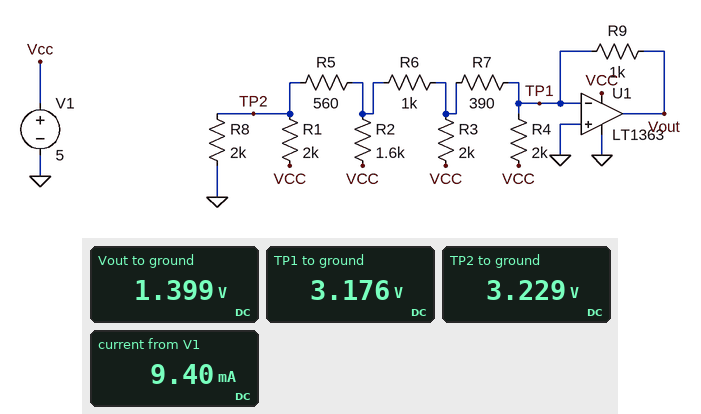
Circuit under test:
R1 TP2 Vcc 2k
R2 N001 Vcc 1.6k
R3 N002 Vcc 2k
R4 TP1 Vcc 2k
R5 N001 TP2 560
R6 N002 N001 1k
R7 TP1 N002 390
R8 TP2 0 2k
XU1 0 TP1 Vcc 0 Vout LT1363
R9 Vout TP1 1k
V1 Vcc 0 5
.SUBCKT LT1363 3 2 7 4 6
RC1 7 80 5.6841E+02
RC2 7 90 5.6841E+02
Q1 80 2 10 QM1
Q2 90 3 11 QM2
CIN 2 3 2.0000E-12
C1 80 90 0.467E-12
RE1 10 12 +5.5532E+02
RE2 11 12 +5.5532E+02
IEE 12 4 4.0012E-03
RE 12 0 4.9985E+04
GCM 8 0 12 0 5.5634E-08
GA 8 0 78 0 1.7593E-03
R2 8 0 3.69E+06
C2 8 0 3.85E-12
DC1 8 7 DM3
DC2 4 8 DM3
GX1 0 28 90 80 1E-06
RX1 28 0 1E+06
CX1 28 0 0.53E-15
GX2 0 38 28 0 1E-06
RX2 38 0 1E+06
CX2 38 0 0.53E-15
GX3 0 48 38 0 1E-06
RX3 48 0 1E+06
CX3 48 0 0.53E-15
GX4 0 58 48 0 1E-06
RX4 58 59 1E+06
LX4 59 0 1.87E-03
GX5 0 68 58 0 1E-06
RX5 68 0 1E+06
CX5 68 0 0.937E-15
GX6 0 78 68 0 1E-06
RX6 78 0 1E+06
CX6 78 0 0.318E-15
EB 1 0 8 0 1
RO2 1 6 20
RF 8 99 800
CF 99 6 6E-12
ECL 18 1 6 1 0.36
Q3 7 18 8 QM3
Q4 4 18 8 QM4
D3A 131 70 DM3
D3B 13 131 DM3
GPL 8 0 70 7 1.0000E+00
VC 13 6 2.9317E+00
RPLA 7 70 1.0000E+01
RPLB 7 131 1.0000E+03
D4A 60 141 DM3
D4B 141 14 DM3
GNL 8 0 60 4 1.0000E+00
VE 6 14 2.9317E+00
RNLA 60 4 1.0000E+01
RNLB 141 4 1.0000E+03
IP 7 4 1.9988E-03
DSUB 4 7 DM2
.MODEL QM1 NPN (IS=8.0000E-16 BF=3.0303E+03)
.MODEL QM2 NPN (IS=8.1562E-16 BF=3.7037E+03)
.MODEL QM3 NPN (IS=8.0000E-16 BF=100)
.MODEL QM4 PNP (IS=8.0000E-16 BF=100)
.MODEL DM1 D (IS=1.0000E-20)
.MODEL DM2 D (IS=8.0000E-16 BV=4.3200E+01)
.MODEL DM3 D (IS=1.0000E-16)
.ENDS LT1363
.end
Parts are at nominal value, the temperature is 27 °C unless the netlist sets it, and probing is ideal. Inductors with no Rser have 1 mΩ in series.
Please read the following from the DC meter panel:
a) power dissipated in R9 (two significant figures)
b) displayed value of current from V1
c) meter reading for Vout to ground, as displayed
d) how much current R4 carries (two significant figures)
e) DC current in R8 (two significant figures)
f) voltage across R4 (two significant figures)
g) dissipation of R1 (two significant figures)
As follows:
3.2 mW
9.40 mA
1.399 V
910 µA
1.6 mA
1.8 V
1.6 mW
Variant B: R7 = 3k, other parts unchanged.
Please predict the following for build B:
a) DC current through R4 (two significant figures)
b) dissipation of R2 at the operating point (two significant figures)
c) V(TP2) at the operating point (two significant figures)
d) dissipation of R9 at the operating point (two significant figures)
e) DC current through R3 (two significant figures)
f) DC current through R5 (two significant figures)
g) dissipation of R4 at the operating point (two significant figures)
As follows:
1.1 mA
840 µW
3.4 V
2.1 mW
510 µA
860 µA
2.3 mW
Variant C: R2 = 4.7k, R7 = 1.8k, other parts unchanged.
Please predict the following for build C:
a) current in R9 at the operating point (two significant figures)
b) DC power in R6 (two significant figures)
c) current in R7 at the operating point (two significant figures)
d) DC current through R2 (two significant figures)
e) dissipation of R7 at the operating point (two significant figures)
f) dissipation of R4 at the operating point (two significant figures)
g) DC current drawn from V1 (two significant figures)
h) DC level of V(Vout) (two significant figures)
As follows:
1.5 mA
60 µW
430 µA
340 µA
330 µW
2.2 mW
9.0 mA
1.4 V
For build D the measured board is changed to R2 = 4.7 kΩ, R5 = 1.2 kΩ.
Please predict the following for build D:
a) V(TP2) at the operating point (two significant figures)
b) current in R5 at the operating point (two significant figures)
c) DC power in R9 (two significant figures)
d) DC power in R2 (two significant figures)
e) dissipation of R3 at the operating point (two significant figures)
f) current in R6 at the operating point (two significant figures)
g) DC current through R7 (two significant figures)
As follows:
2.9 V
390 µA
2.9 mW
570 µW
1.3 mW
41 µA
760 µA
